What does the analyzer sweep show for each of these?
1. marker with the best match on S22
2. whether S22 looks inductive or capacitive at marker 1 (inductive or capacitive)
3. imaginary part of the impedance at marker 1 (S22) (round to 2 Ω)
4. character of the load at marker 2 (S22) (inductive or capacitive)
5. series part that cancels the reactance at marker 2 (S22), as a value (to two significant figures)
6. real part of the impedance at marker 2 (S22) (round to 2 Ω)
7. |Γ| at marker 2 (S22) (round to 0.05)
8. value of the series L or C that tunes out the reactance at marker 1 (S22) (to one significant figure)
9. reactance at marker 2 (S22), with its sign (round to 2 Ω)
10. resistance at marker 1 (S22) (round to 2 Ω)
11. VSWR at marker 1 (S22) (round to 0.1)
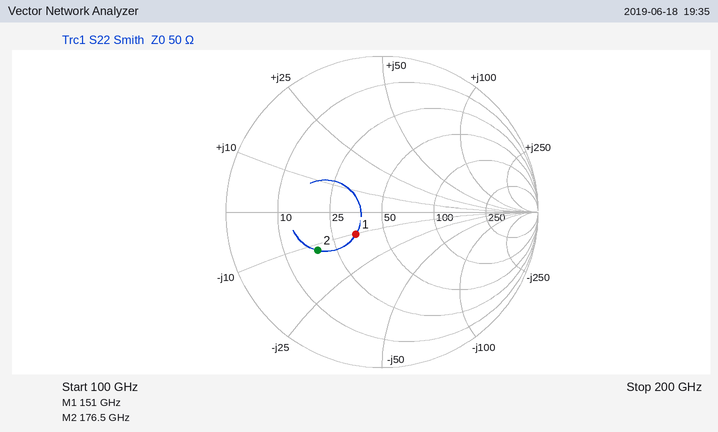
marker 1
capacitive
-10 Ω
capacitive
11 pH
18 Ω
0.50
10 pH
-12 Ω
34 Ω
1.6
